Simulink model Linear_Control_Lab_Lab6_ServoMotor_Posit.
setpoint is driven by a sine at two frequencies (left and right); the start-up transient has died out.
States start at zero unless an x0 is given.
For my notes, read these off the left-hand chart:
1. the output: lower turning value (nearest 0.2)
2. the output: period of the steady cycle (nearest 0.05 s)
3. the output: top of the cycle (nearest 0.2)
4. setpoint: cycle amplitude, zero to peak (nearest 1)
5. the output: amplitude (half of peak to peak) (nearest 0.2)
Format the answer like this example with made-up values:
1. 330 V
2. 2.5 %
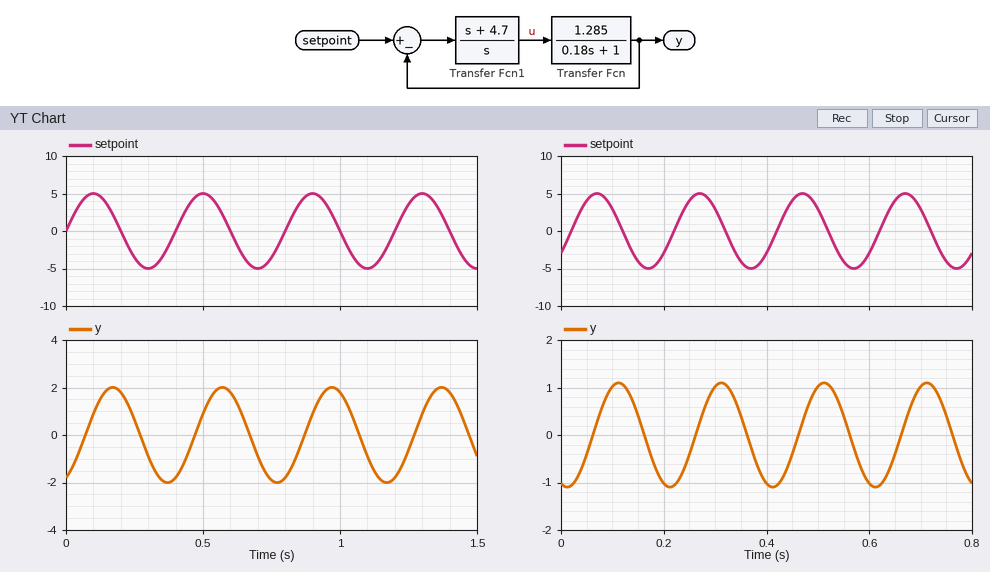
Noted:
1. -2.0
2. 0.40 s
3. 2.0
4. 5
5. 2.0
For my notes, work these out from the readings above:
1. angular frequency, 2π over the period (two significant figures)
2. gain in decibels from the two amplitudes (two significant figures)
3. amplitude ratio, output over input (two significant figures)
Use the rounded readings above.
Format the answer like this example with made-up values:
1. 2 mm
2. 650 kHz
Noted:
1. 16 rad/s
2. -8.0 dB
3. 0.40
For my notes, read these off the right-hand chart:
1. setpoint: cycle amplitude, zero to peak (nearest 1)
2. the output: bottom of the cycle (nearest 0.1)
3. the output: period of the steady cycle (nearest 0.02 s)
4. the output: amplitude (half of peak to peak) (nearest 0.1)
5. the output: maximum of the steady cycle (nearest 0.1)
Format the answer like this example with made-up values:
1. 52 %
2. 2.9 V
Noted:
1. 5
2. -1.1
3. 0.20 s
4. 1.1
5. 1.1
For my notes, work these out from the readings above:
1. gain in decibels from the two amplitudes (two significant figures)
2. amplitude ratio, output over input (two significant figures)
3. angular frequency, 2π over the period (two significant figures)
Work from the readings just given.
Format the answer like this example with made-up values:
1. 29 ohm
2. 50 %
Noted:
1. -13 dB
2. 0.22
3. 31 rad/s
